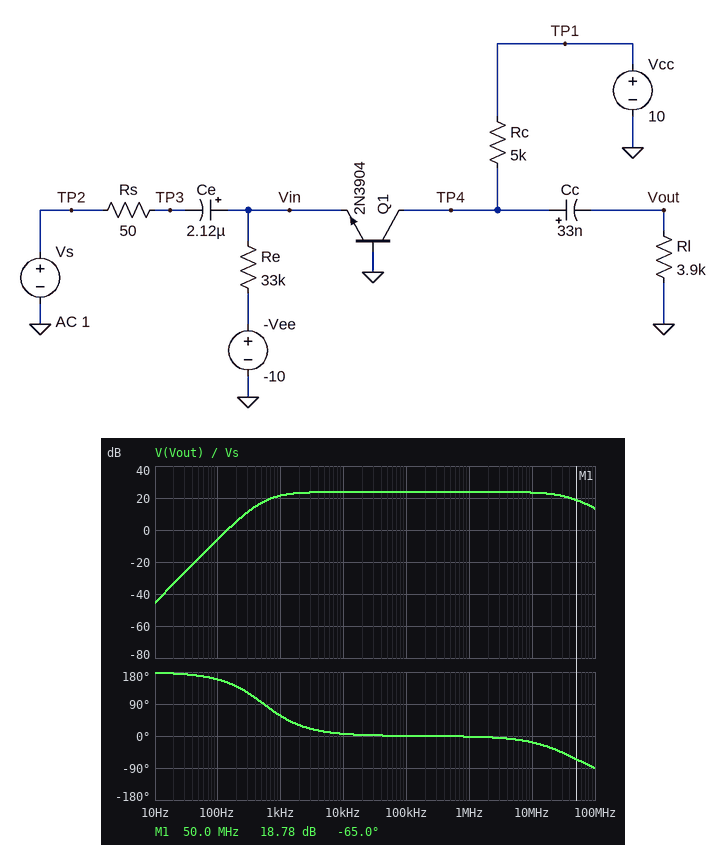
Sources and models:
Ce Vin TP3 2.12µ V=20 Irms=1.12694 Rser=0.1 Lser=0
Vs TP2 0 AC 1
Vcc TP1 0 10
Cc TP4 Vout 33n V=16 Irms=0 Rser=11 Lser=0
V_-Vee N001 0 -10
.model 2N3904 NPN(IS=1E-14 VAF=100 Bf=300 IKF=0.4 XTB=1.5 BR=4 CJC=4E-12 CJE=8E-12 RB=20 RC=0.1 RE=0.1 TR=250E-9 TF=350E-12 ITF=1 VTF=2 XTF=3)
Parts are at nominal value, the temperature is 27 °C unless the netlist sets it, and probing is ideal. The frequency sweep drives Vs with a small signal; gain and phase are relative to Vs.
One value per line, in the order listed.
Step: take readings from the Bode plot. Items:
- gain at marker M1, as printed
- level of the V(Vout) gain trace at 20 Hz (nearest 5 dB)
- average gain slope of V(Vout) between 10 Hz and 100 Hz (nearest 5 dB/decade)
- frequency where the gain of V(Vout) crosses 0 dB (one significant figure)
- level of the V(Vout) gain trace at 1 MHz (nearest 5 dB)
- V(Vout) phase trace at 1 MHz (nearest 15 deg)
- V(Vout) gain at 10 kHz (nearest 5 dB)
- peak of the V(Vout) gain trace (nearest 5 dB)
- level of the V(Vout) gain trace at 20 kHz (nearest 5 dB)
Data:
18.78 dB
-35 dB
40 dB/decade
100 Hz
25 dB
0 deg
25 dB
25 dB
25 dB
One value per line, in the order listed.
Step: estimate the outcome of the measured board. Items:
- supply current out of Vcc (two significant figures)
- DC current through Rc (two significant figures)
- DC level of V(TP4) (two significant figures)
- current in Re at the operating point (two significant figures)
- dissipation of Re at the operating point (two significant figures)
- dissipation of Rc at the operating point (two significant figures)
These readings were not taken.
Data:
280 µA
280 µA
8.6 V
280 µA
2.7 mW
400 µW
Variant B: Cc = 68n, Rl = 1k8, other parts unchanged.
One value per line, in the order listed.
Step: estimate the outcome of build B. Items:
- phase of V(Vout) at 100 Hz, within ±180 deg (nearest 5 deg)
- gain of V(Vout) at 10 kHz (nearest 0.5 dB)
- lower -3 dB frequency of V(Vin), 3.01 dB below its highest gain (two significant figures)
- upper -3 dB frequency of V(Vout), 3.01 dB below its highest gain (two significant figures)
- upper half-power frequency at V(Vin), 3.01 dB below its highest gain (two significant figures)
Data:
155 deg
19.5 dB
540 Hz
54 MHz
360 MHz
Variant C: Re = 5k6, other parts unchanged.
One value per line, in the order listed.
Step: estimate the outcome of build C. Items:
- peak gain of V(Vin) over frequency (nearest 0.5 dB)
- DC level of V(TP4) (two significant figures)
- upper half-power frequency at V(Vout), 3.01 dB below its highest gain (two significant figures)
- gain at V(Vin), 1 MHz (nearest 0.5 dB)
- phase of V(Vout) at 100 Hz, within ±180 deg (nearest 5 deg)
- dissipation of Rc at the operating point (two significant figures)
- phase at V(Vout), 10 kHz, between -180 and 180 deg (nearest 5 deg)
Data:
-8.0 dB
1.7 V
20 MHz
-12.0 dB
165 deg
14 mW
10 deg
